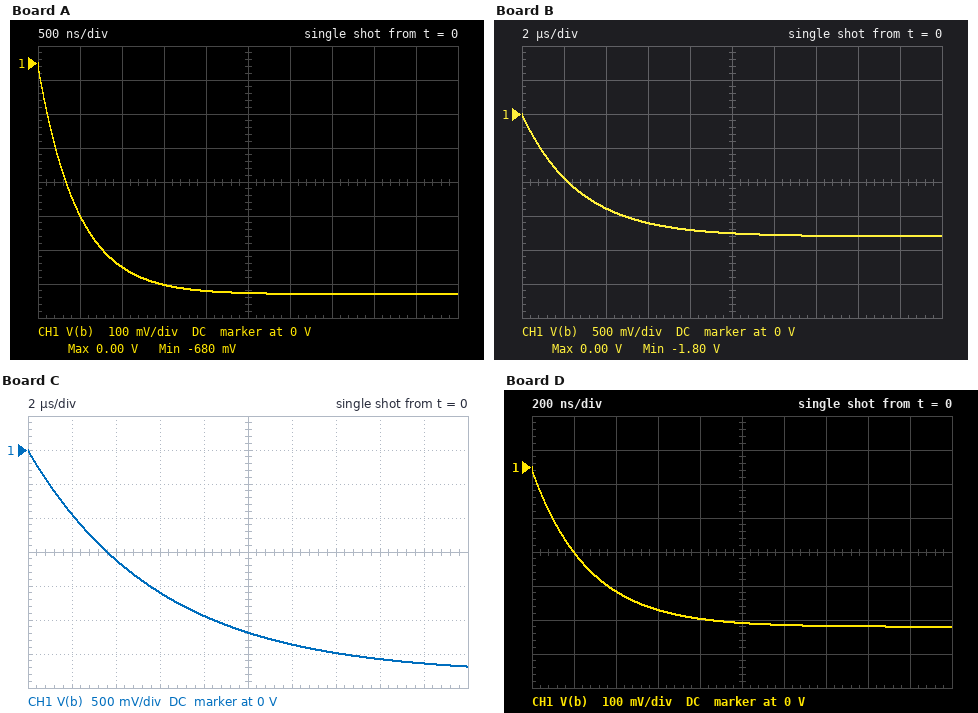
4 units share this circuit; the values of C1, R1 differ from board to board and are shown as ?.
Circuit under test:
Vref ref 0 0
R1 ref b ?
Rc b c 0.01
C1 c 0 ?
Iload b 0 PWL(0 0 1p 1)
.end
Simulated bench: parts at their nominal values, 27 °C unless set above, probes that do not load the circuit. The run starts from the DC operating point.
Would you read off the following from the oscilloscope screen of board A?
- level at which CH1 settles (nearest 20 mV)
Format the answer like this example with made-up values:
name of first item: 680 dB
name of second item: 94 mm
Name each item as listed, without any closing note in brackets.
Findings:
level at which CH1 settles: -680 mV
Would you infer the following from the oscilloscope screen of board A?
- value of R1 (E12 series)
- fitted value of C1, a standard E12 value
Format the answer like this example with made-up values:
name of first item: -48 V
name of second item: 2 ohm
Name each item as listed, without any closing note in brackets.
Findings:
value of R1: 0.68 Ω
fitted value of C1, a standard E12 value: 680 nF
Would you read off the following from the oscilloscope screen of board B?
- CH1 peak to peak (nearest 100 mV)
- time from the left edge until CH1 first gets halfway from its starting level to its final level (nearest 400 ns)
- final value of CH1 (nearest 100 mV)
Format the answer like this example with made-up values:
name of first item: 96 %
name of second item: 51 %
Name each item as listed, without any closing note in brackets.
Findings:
CH1 peak to peak: 1.8 V
time from the left edge until CH1 first gets halfway from its starting level to its final level: 2.0 µs
final value of CH1: -1.8 V
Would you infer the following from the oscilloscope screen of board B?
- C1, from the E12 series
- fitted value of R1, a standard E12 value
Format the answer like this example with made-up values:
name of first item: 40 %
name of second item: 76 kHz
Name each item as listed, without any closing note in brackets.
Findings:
C1, from the E12 series: 1.5 µF
fitted value of R1, a standard E12 value: 1.8 Ω
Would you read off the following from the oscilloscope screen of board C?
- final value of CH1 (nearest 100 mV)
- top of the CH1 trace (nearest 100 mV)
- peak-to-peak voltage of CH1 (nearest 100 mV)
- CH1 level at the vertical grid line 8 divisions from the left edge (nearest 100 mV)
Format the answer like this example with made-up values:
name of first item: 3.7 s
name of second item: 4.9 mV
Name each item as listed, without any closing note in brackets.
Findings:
final value of CH1: -3.2 V
top of the CH1 trace: 0 V
peak-to-peak voltage of CH1: 3.2 V
CH1 level at the vertical grid line 8 divisions from the left edge: -3.1 V
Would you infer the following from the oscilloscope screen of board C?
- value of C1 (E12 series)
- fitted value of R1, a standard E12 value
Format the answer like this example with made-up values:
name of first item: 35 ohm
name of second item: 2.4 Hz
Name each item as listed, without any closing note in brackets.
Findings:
value of C1: 1.8 µF
fitted value of R1, a standard E12 value: 3.3 Ω
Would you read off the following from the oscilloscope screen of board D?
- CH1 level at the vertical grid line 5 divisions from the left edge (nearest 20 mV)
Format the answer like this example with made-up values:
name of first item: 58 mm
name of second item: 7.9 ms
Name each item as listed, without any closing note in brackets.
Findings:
CH1 level at the vertical grid line 5 divisions from the left edge: -460 mV
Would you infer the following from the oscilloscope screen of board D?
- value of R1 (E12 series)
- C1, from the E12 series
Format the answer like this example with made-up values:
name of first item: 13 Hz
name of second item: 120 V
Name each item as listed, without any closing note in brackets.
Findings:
value of R1: 0.47 Ω
C1, from the E12 series: 560 nF
